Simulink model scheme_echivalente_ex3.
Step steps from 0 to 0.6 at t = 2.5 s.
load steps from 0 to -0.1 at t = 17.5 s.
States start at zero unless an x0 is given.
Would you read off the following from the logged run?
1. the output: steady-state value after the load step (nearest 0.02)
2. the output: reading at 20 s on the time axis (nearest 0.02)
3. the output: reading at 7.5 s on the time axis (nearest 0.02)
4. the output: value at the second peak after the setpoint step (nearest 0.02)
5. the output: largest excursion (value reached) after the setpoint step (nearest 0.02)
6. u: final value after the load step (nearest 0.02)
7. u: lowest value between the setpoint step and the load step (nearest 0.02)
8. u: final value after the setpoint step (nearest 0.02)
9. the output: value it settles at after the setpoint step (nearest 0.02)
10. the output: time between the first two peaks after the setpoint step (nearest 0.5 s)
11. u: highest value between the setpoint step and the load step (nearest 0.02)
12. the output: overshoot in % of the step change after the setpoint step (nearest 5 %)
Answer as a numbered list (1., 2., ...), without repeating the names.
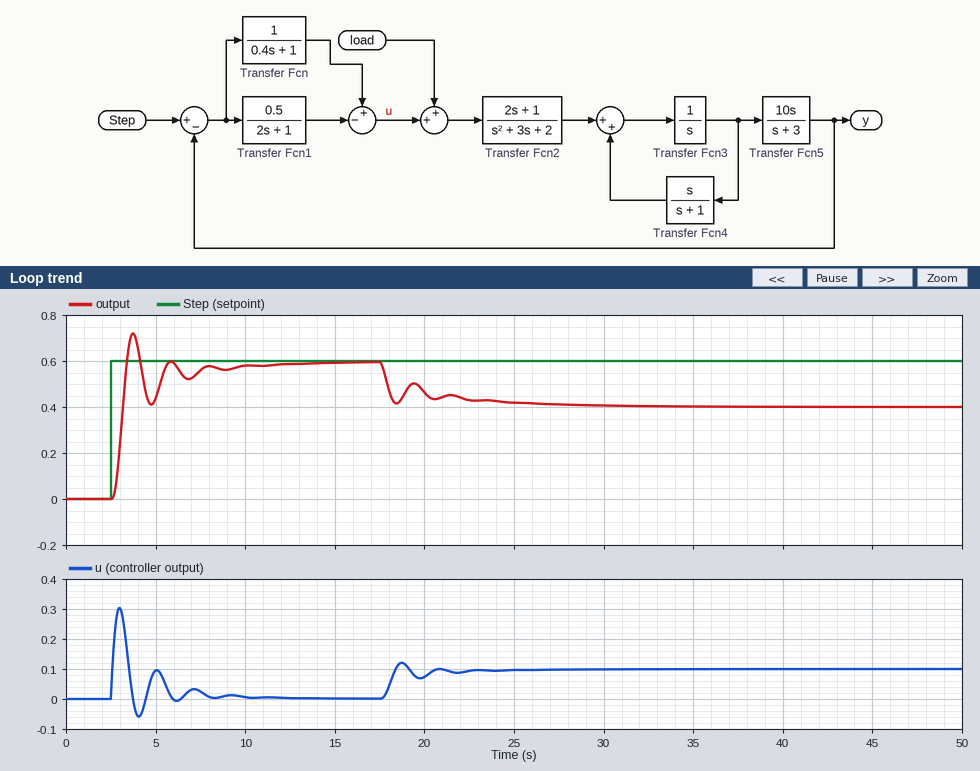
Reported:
1. 0.40
2. 0.46
3. 0.56
4. 0.60
5. 0.72
6. 0.10
7. -0.06
8. 0.00
9. 0.60
10. 2.0 s
11. 0.30
12. 20 %
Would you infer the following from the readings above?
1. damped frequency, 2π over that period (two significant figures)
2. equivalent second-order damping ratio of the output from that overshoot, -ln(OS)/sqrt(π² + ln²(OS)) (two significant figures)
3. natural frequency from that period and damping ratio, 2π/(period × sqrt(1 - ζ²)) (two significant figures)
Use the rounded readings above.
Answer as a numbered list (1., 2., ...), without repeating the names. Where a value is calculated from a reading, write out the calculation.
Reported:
1. 2π / 2 = 3.1 rad/s
2. ln(0.2) = -1.609; 1.609 / sqrt(9.870 + 2.590) = 0.46
3. 2π / (2 × sqrt(1 - 0.46²)) = 3.5 rad/s
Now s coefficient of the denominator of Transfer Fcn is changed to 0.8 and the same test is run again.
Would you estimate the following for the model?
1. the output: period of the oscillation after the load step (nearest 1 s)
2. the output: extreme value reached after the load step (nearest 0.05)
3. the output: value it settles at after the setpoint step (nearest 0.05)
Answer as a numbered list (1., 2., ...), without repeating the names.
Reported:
1. 3 s
2. 0.35
3. 0.60
